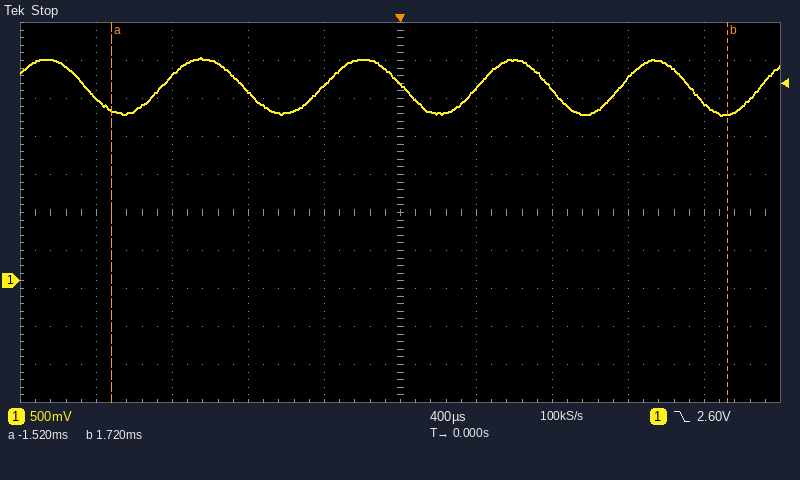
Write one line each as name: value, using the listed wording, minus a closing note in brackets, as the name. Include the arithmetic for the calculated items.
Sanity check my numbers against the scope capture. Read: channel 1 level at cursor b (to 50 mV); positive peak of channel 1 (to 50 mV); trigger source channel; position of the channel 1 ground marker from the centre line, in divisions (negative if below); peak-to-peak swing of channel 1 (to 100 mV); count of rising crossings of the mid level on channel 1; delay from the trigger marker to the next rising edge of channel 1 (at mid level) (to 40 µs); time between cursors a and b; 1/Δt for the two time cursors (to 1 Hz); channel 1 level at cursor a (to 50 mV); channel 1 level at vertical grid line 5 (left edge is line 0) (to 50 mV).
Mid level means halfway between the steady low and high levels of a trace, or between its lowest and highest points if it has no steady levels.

channel 1 level at cursor b: 2.20 V
positive peak of channel 1: 2.95 V
trigger source channel: channel 1
position of the channel 1 ground marker from the centre line, in divisions: -1.8 div
peak-to-peak swing of channel 1: 800 mV
count of rising crossings of the mid level on channel 1: 5
delay from the trigger marker to the next rising edge of channel 1 (at mid level): 400 µs
time between cursors a and b: 1.72 ms − (-1.52 ms) = 3.24 ms
1/Δt for the two time cursors: 1 / 3.24 ms ≈ 309 Hz
channel 1 level at cursor a: 2.25 V
channel 1 level at vertical grid line 5 (left edge is line 0): 2.60 V
